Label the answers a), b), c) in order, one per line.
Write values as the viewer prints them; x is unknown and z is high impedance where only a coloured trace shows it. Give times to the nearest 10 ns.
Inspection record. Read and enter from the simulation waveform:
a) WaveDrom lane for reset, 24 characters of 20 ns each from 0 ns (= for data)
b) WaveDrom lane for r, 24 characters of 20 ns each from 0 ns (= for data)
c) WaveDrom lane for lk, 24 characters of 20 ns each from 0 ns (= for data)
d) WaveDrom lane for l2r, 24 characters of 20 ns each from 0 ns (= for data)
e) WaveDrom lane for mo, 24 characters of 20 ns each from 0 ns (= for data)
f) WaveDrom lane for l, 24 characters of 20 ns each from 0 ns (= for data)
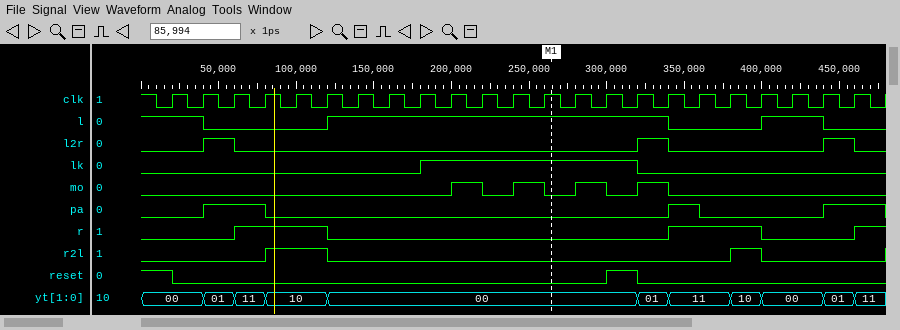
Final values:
a) {name: 'reset', wave: '10.............10.......'}
b) {name: 'r', wave: '0..1..0..........1..0..1'}
c) {name: 'lk', wave: '0........1......0.......'}
d) {name: 'l2r', wave: '0.10............10....10'}
e) {name: 'mo', wave: '0.........10101010......'}
f) {name: 'l', wave: '1.0...1..........0..1.0.'}
